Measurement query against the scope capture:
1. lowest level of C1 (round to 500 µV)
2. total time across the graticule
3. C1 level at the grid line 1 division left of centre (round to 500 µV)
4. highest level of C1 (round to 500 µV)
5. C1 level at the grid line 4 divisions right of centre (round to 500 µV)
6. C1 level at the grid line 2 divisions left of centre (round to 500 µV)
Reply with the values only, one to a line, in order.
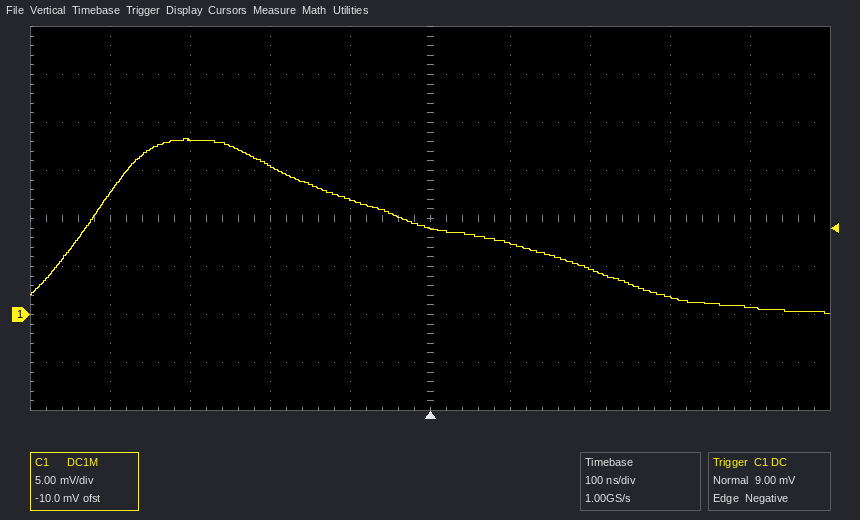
0.0 mV
1 µs
12.0 mV
18.5 mV
500 µV
15.5 mV
